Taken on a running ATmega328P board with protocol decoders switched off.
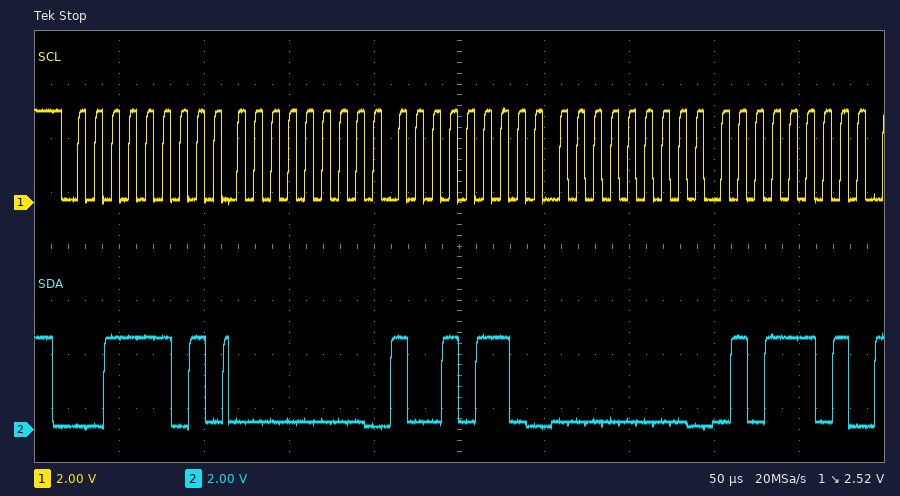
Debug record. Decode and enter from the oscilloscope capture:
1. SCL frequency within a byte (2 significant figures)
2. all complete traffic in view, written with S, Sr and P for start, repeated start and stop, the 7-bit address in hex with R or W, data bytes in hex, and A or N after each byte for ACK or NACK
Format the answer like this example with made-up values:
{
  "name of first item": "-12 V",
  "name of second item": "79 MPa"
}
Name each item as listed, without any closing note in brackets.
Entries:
{
  "SCL frequency within a byte": "100 kHz",
  "all complete traffic in view, written with S, Sr and P for start, repeated start and stop, the 7-bit address in hex with R or W, data bytes in hex, and A or N after each byte for ACK or NACK": "S 1ER A 00 A 96 A 00 A 5D A"
}
